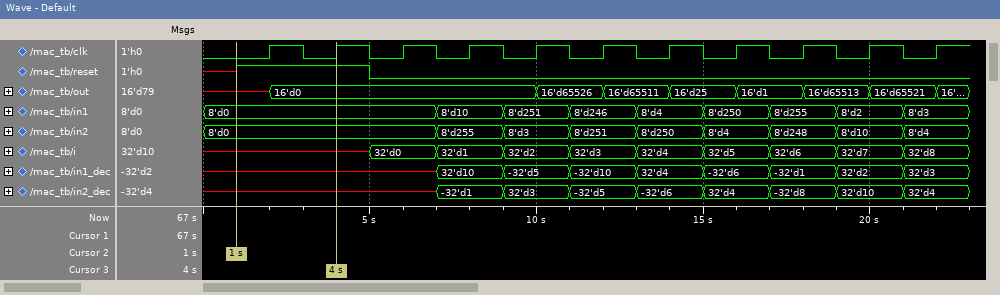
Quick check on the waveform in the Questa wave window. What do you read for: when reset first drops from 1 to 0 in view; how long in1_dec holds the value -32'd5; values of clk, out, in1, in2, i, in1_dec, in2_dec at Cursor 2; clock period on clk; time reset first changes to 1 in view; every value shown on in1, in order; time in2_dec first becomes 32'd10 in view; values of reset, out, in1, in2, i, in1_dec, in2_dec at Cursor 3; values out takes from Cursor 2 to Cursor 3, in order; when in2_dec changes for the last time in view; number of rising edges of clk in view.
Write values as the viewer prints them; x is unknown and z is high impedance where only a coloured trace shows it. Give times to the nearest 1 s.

5 s
2 s
clk=0, out=x, in1=8'd0, in2=8'd0, i=x, in1_dec=x, in2_dec=x
2 s
1 s
8'd0, 8'd10, 8'd251, 8'd246, 8'd4, 8'd250, 8'd255, 8'd2, 8'd3
19 s
reset=1, out=16'd0, in1=8'd0, in2=8'd0, i=x, in1_dec=x, in2_dec=x
x, 16'd0
21 s
11
